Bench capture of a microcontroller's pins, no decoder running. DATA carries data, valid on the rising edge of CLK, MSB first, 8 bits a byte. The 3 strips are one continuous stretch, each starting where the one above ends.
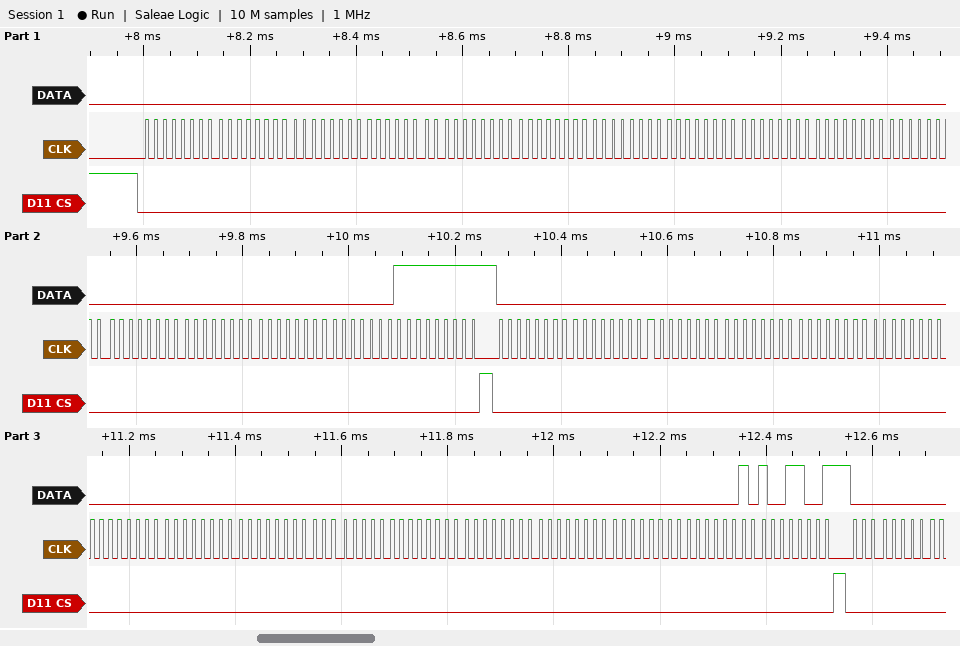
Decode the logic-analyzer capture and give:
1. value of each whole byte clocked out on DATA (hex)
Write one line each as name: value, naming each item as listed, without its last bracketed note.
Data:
value of each whole byte clocked out on DATA: 00 00 00 00 00 00 00 00 00 00 00 00 00 00 01 FF 00 00 00 00 00 00 00 00 00 00 00 00 00 00 02 99 00
